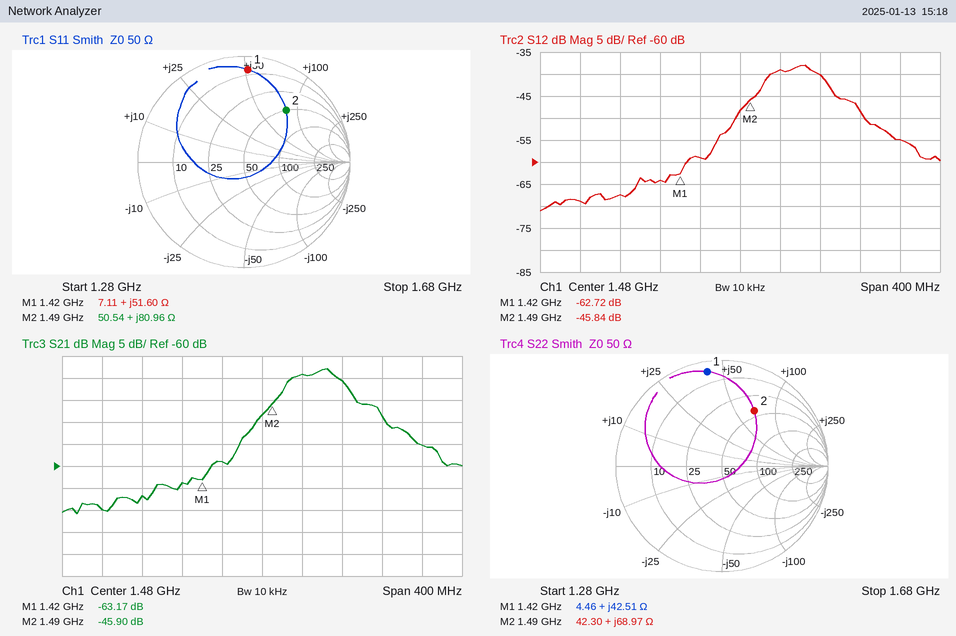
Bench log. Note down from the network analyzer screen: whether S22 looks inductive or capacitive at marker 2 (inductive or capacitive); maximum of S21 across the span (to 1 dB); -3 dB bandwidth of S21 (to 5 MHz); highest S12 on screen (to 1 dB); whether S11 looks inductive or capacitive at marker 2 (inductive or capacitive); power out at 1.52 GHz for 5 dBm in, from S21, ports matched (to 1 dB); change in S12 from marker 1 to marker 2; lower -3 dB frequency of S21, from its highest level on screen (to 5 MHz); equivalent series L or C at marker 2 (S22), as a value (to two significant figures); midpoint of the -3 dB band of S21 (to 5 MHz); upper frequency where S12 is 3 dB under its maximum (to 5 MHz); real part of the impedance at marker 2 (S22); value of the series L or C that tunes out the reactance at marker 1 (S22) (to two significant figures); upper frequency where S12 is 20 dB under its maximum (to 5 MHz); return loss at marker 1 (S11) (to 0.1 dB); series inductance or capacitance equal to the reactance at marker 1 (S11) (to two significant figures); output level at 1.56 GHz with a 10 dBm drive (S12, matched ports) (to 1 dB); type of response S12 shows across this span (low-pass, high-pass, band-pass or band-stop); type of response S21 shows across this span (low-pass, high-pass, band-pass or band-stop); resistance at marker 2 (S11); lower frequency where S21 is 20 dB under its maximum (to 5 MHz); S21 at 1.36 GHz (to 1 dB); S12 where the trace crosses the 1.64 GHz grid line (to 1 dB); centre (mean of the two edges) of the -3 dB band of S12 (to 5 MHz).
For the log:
inductive
-38 dB
55 MHz
-38 dB
inductive
-34 dBm
16.88 dB
1.505 GHz
7.4 nH
1.535 GHz
1.565 GHz
42.30 Ω
2.6 pF
1.660 GHz
1.2 dB
5.8 nH
-30 dBm
band-pass
band-pass
50.54 Ω
1.450 GHz
-67 dB
-55 dB
1.535 GHz
